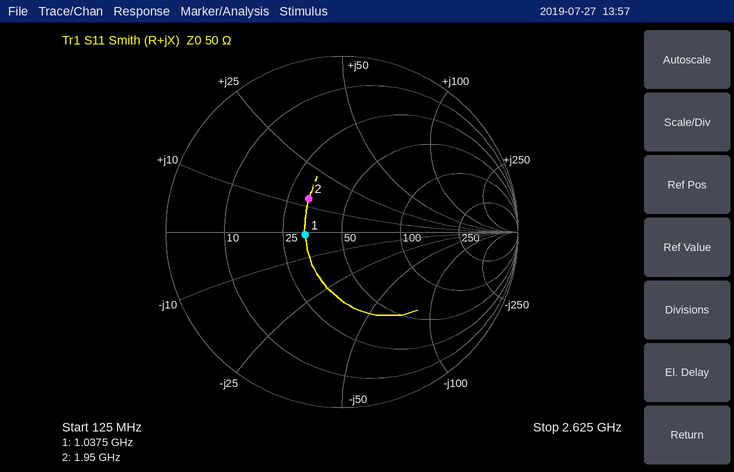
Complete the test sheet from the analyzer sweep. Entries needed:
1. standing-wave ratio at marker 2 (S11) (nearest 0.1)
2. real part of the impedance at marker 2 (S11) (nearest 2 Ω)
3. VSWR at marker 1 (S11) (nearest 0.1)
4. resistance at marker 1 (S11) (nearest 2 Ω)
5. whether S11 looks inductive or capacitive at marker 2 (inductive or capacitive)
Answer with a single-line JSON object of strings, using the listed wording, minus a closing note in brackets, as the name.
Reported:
{"standing-wave ratio at marker 2 (S11)": "1.7", "real part of the impedance at marker 2 (S11)": "32 Ω", "VSWR at marker 1 (S11)": "1.5", "resistance at marker 1 (S11)": "32 Ω", "whether S11 looks inductive or capacitive at marker 2": "inductive"}
